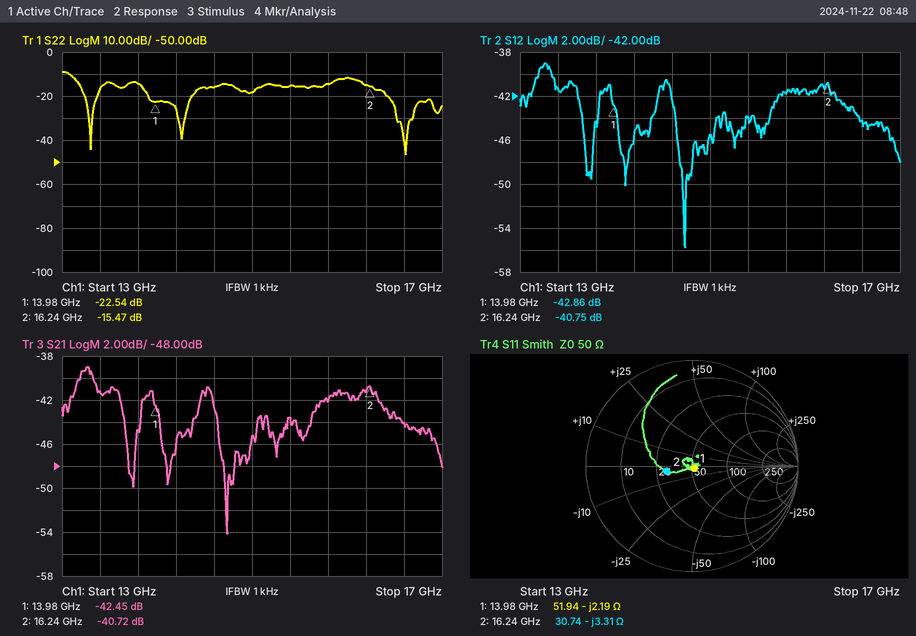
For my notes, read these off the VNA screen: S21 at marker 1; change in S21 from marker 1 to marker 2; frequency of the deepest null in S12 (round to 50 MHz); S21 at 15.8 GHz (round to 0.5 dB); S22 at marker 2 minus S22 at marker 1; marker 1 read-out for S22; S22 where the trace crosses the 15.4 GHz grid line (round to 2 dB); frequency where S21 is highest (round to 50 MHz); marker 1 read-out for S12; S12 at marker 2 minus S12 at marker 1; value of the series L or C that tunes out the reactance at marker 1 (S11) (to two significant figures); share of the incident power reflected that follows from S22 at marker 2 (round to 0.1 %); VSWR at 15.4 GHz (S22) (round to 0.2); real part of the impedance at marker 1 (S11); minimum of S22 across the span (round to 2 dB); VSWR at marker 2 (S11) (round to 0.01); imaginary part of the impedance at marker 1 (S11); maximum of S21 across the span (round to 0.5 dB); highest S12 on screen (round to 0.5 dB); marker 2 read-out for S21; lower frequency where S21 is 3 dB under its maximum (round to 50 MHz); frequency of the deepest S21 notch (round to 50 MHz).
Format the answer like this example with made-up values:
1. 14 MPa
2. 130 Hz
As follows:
1. -42.45 dB
2. 1.73 dB
3. 14.75 GHz
4. -42.0 dB
5. 7.07 dB
6. -22.54 dB
7. -16 dB
8. 13.25 GHz
9. -42.86 dB
10. 2.11 dB
11. 25 pH
12. 2.8 %
13. 1.4
14. 51.94 Ω
15. -46 dB
16. 1.64
17. -2.19 Ω
18. -39.0 dB
19. -39.0 dB
20. -40.72 dB
21. 13.10 GHz
22. 14.75 GHz
